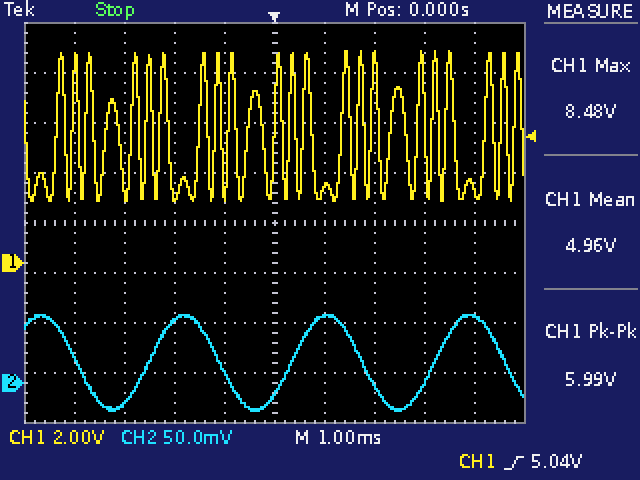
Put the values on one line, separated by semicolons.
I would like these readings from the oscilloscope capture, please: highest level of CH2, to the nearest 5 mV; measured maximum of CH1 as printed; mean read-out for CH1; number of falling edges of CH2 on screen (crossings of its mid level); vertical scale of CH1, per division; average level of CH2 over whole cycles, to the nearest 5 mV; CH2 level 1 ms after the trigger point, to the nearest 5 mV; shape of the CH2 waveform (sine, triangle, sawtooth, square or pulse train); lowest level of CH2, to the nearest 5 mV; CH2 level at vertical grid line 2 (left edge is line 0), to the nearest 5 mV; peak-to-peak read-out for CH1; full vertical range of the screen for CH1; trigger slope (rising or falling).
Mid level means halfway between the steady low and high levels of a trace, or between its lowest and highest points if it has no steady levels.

70 mV; 8.48 V; 4.96 V; 4; 2 V; 20 mV; 65 mV; sine; -30 mV; -20 mV; 5.99 V; 16 V; rising
